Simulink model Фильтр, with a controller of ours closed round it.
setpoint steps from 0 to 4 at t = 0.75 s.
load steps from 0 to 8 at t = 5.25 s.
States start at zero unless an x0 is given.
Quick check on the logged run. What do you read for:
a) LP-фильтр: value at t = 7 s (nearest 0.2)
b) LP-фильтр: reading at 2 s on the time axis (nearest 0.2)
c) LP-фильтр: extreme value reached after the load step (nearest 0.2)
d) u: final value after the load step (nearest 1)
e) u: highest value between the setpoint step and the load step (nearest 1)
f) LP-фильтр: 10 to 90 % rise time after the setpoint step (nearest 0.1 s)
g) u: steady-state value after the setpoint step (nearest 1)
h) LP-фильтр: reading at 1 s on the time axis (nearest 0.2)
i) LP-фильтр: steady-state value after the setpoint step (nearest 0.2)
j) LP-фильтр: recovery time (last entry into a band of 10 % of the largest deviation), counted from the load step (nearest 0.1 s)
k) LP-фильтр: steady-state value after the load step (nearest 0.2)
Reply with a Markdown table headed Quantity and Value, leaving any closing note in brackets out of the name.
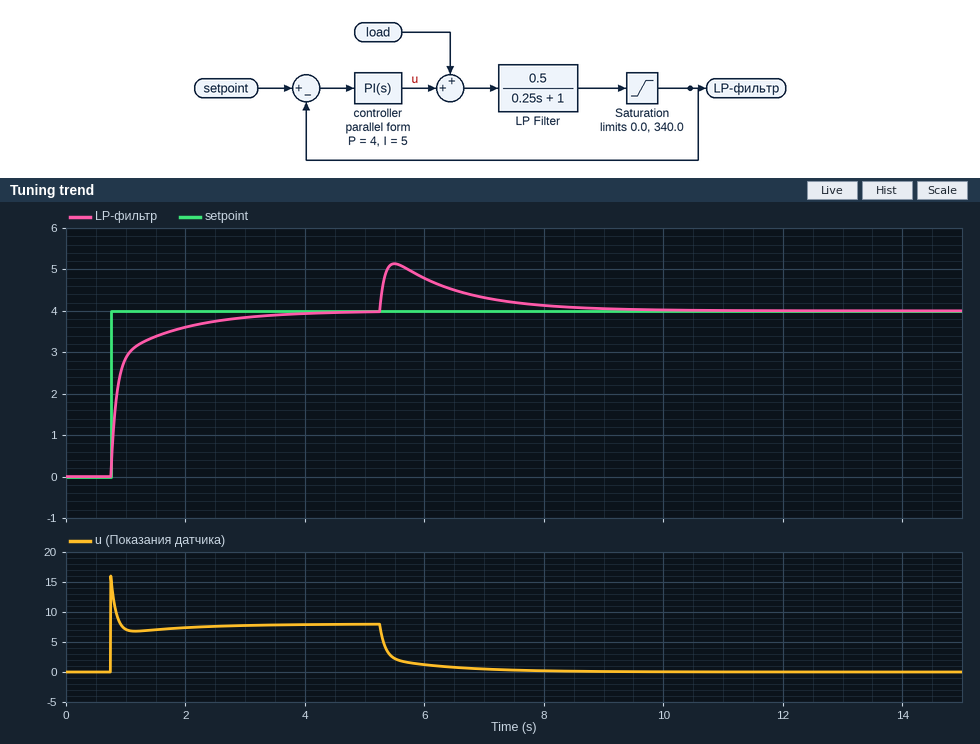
| Quantity | Value |
|---|---|
| LP-фильтр: value at t = 7 s | 4.4 |
| LP-фильтр: reading at 2 s on the time axis | 3.6 |
| LP-фильтр: extreme value reached after the load step | 5.2 |
| u: final value after the load step | 0 |
| u: highest value between the setpoint step and the load step | 16 |
| LP-фильтр: 10 to 90 % rise time after the setpoint step | 1.2 s |
| u: steady-state value after the setpoint step | 8 |
| LP-фильтр: reading at 1 s on the time axis | 2.8 |
| LP-фильтр: steady-state value after the setpoint step | 4.0 |
| LP-фильтр: recovery time (last entry into a band of 10 % of the largest deviation), counted from the load step | 2.9 s |
| LP-фильтр: steady-state value after the load step | 4.0 |
